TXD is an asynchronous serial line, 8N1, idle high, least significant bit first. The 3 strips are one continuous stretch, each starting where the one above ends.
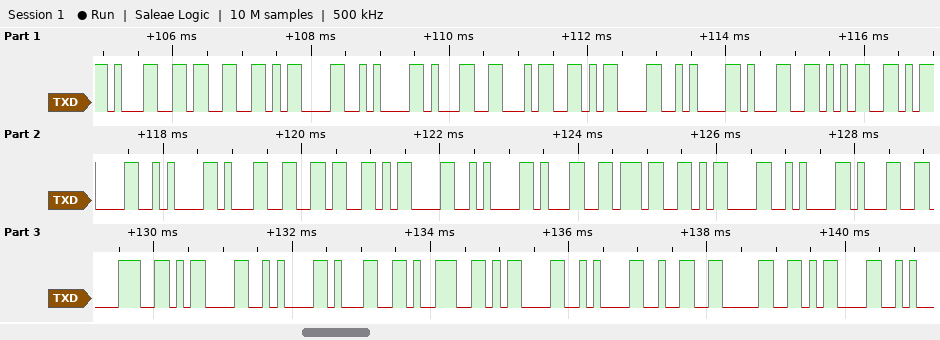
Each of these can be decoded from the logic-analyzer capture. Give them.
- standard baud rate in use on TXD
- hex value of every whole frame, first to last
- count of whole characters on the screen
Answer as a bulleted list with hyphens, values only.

- 9600 baud
- 31 33 0D 0A 31 34 0D 0A 31 35 0D 0A 31 36 0D 0A 31 37 0D 0A 31 38 0D 0A 31 39 0D 0A 32 30 0D
- 31
